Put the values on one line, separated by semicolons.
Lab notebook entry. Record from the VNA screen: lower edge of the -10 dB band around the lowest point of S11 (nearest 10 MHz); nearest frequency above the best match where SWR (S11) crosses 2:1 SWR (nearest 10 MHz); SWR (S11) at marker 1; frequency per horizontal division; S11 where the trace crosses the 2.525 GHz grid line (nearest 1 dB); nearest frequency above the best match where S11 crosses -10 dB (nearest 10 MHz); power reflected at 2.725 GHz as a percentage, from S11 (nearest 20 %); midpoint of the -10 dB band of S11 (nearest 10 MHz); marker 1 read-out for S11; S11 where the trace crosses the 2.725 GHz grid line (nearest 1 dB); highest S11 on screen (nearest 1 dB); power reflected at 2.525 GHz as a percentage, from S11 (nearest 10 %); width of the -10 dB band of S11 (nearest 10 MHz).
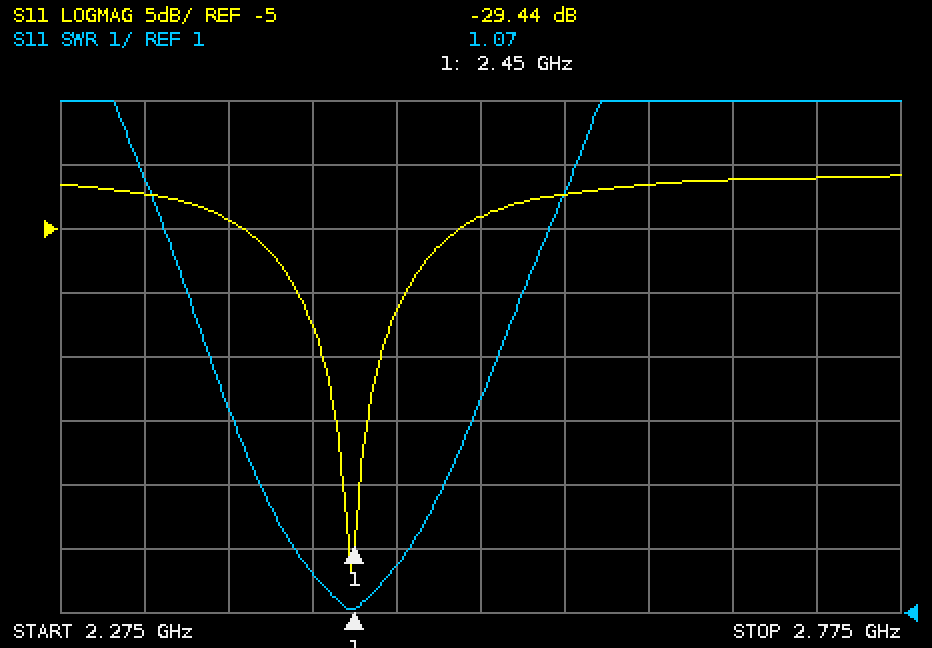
2.42 GHz; 2.48 GHz; 1.07; 50 MHz; -4 dB; 2.48 GHz; 80 %; 2.45 GHz; -29.44 dB; -1 dB; -1 dB; 40 %; 60 MHz
